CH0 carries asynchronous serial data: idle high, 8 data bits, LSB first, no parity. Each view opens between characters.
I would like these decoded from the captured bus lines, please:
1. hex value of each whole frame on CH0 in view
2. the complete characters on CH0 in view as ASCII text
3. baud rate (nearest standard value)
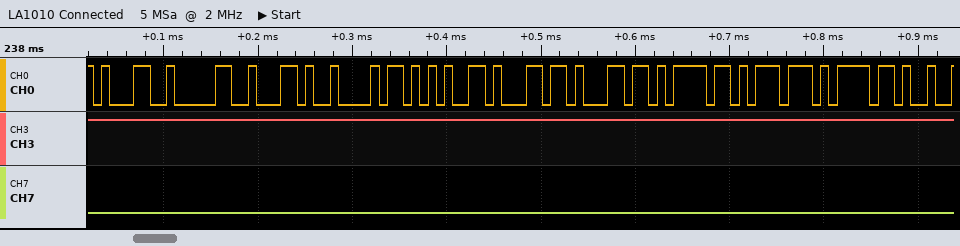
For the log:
31, 30, 2C, 68, 65, 6C, 6C, 6F, 77, 6F
"10,hellowo"
115200 baud
